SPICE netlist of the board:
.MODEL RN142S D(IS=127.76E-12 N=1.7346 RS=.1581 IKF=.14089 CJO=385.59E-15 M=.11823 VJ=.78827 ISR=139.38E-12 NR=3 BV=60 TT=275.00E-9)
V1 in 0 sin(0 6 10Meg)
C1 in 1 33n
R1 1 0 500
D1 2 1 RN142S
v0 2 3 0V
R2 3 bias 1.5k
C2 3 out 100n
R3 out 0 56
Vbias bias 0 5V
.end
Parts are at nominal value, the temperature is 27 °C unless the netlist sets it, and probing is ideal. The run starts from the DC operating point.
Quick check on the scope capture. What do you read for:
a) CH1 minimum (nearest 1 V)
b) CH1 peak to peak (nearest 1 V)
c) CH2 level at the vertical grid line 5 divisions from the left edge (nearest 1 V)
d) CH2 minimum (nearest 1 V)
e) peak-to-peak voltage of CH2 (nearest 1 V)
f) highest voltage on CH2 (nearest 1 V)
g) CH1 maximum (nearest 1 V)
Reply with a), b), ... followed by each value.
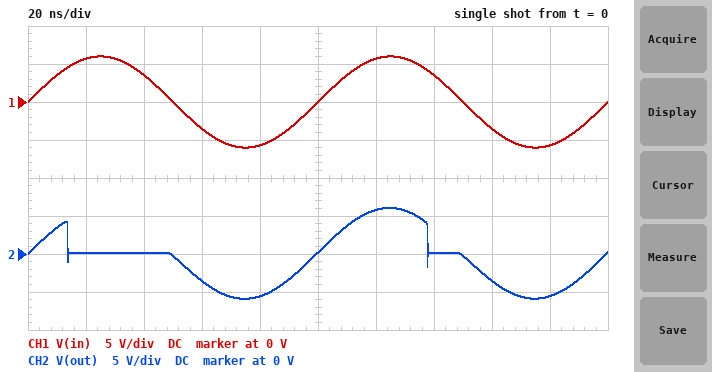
a) -6 V
b) 12 V
c) 0 V
d) -6 V
e) 12 V
f) 6 V
g) 6 V
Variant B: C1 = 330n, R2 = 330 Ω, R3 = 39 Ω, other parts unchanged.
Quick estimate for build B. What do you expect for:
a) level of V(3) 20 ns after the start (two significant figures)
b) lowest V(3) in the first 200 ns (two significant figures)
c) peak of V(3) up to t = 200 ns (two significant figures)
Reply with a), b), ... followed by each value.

a) 3.5 V
b) -2.6 V
c) 9.3 V
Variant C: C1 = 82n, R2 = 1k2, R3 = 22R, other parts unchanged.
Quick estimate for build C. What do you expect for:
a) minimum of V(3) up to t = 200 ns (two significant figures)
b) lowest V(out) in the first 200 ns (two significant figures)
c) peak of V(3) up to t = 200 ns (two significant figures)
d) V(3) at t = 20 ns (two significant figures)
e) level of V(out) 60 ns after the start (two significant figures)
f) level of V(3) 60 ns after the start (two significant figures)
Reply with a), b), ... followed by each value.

a) -3.8 V
b) -5.8 V
c) 8.1 V
d) 2.1 V
e) -3.5 V
f) -1.5 V
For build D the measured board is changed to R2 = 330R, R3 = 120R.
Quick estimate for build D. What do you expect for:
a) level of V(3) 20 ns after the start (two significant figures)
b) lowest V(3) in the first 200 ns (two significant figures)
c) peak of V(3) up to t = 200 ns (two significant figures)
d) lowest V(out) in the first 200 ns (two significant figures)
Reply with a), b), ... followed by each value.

a) 9.0 V
b) -2.7 V
c) 9.3 V
d) -6.0 V
